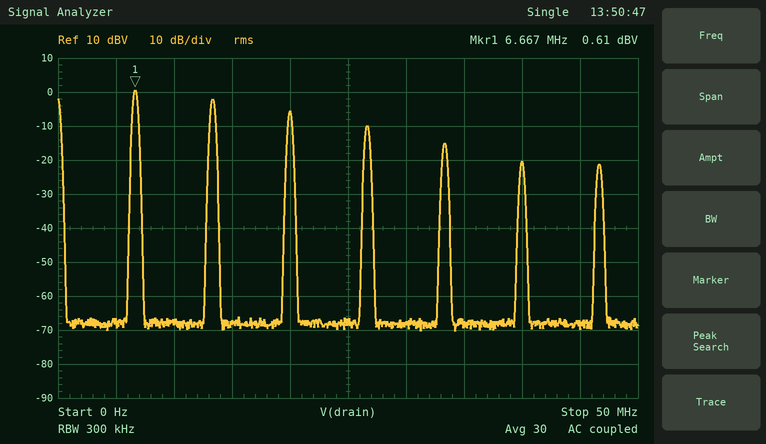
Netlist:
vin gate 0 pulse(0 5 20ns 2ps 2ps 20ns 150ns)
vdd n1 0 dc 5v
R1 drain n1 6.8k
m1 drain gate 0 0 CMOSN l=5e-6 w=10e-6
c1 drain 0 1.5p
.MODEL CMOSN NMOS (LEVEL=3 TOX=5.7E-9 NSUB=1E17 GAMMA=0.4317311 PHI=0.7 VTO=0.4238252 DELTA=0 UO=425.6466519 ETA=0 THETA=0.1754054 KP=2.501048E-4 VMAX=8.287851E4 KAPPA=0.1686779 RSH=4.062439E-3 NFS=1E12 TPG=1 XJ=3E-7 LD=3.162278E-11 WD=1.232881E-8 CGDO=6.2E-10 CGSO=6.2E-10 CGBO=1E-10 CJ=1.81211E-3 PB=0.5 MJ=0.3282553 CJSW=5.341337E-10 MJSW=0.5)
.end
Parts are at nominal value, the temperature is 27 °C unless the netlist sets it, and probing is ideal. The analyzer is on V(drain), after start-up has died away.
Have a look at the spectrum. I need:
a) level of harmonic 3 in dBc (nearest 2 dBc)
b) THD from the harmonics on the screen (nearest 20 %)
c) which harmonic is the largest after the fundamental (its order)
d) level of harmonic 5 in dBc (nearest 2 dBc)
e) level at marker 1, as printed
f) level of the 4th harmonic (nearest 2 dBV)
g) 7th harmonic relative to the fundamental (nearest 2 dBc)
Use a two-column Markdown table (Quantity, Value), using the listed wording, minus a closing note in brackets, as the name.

| Quantity | Value |
|---|---|
| level of harmonic 3 in dBc | -6 dBc |
| THD from the harmonics on the screen | 100 % |
| which harmonic is the largest after the fundamental | 2 |
| level of harmonic 5 in dBc | -16 dBc |
| level at marker 1, as printed | 0.61 dBV |
| level of the 4th harmonic | -10 dBV |
| 7th harmonic relative to the fundamental | -22 dBc |
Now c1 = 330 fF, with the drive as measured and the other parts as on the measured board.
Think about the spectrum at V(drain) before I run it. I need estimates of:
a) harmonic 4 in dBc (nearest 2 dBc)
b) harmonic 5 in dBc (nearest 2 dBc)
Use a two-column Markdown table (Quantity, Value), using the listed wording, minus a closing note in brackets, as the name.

| Quantity | Value |
|---|---|
| harmonic 4 in dBc | -6 dBc |
| harmonic 5 in dBc | -10 dBc |
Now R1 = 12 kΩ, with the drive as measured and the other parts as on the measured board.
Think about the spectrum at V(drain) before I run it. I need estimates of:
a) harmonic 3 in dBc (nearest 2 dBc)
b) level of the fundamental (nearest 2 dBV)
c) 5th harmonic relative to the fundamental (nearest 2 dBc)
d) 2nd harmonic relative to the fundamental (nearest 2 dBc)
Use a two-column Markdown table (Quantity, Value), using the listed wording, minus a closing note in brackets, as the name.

| Quantity | Value |
|---|---|
| harmonic 3 in dBc | -8 dBc |
| level of the fundamental | 2 dBV |
| 5th harmonic relative to the fundamental | -18 dBc |
| 2nd harmonic relative to the fundamental | -4 dBc |
